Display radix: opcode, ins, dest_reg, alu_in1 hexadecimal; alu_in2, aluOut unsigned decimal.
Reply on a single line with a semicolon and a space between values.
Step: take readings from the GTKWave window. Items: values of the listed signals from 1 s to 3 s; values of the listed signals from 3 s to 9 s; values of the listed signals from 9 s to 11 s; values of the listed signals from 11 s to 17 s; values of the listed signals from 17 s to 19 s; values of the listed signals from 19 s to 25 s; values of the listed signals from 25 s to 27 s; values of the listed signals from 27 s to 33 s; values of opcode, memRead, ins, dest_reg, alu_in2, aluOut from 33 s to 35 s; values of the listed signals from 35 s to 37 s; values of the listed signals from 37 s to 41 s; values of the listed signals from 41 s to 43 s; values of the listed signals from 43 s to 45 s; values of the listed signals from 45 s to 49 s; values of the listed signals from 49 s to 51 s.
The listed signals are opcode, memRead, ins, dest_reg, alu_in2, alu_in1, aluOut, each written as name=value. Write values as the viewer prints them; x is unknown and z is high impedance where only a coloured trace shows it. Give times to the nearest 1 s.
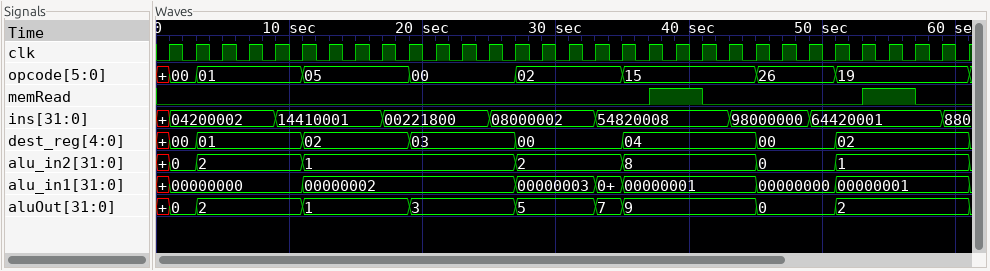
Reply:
opcode=00, memRead=0, ins=04200002, dest_reg=00, alu_in2=0, alu_in1=00000000, aluOut=0; opcode=01, memRead=0, ins=04200002, dest_reg=01, alu_in2=2, alu_in1=00000000, aluOut=2; opcode=01, memRead=0, ins=14410001, dest_reg=01, alu_in2=2, alu_in1=00000000, aluOut=2; opcode=05, memRead=0, ins=14410001, dest_reg=02, alu_in2=1, alu_in1=00000002, aluOut=1; opcode=05, memRead=0, ins=00221800, dest_reg=02, alu_in2=1, alu_in1=00000002, aluOut=1; opcode=00, memRead=0, ins=00221800, dest_reg=03, alu_in2=1, alu_in1=00000002, aluOut=3; opcode=00, memRead=0, ins=08000002, dest_reg=03, alu_in2=1, alu_in1=00000002, aluOut=3; opcode=02, memRead=0, ins=08000002, dest_reg=00, alu_in2=2, alu_in1=00000003, aluOut=5; opcode=02, memRead=0, ins=54820008, dest_reg=00, alu_in2=2, aluOut=7; opcode=15, memRead=0, ins=54820008, dest_reg=04, alu_in2=8, alu_in1=00000001, aluOut=9; opcode=15, memRead=1, ins=54820008, dest_reg=04, alu_in2=8, alu_in1=00000001, aluOut=9; opcode=15, memRead=0, ins=54820008, dest_reg=04, alu_in2=8, alu_in1=00000001, aluOut=9; opcode=15, memRead=0, ins=98000000, dest_reg=04, alu_in2=8, alu_in1=00000001, aluOut=9; opcode=26, memRead=0, ins=98000000, dest_reg=00, alu_in2=0, alu_in1=00000000, aluOut=0; opcode=26, memRead=0, ins=64420001, dest_reg=00, alu_in2=0, alu_in1=00000000, aluOut=0
